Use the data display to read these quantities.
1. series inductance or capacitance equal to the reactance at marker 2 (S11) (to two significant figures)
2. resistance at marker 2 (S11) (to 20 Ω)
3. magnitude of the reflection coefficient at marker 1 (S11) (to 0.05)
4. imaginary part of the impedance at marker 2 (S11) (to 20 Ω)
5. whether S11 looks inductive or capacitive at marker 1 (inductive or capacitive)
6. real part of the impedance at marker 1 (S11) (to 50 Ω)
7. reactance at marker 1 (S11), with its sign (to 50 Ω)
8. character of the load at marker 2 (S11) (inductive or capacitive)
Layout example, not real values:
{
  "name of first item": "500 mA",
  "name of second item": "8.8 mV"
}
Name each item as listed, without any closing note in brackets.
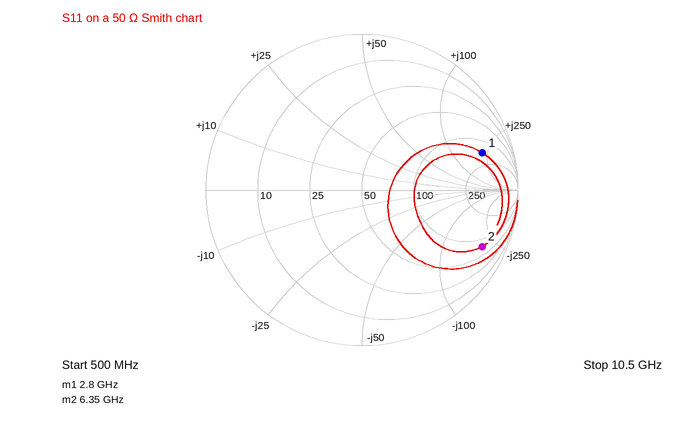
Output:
{
  "series inductance or capacitance equal to the reactance at marker 2 (S11)": "130 fF",
  "resistance at marker 2 (S11)": "80 Ω",
  "magnitude of the reflection coefficient at marker 1 (S11)": "0.80",
  "imaginary part of the impedance at marker 2 (S11)": "-200 Ω",
  "whether S11 looks inductive or capacitive at marker 1": "inductive",
  "real part of the impedance at marker 1 (S11)": "150 Ω",
  "reactance at marker 1 (S11), with its sign": "+200 Ω",
  "character of the load at marker 2 (S11)": "capacitive"
}
